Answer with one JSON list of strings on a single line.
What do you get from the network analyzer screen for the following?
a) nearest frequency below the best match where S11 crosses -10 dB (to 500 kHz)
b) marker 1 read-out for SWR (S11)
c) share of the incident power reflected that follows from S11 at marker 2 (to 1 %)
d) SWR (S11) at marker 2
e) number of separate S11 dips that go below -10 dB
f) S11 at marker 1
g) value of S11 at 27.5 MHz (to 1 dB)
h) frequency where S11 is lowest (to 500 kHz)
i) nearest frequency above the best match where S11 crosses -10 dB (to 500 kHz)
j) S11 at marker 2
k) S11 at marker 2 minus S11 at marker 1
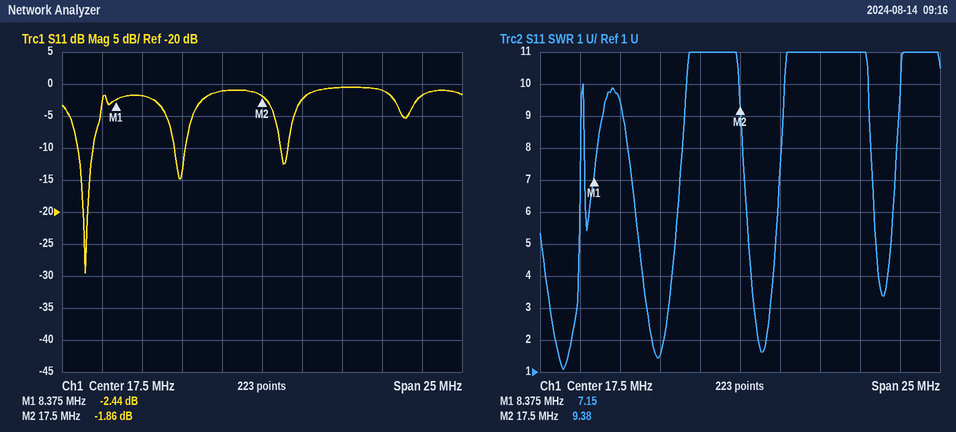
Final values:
["6.0 MHz", "7.15", "65 %", "9.38", "3", "-2.44 dB", "-2 dB", "6.5 MHz", "7.0 MHz", "-1.86 dB", "0.58 dB"]
